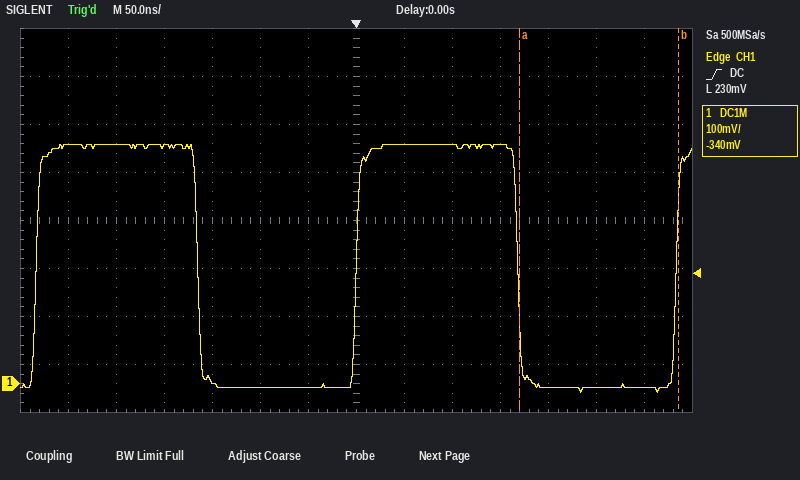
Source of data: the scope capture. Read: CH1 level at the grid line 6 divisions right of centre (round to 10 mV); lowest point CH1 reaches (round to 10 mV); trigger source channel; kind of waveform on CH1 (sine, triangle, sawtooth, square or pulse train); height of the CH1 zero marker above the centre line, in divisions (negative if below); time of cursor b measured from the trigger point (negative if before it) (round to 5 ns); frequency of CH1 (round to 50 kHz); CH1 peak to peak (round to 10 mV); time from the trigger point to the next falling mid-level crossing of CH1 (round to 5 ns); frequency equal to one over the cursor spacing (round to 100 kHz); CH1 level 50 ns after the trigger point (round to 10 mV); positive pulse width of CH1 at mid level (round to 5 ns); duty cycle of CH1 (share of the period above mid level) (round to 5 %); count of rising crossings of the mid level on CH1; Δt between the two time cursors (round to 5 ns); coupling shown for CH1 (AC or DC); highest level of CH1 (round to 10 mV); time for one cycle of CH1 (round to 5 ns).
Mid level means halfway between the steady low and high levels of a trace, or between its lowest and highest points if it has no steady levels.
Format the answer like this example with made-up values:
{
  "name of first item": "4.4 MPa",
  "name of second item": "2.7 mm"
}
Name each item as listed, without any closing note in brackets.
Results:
{
  "CH1 level at the grid line 6 divisions right of centre": "-10 mV",
  "lowest point CH1 reaches": "-20 mV",
  "trigger source channel": "CH1",
  "kind of waveform on CH1": "square",
  "height of the CH1 zero marker above the centre line, in divisions": "-3.4 div",
  "time of cursor b measured from the trigger point (negative if before it)": "+335 ns",
  "frequency of CH1": "3.00 MHz",
  "CH1 peak to peak": "520 mV",
  "time from the trigger point to the next falling mid-level crossing of CH1": "170 ns",
  "frequency equal to one over the cursor spacing": "6.1 MHz",
  "CH1 level 50 ns after the trigger point": "500 mV",
  "positive pulse width of CH1 at mid level": "170 ns",
  "duty cycle of CH1 (share of the period above mid level)": "50 %",
  "count of rising crossings of the mid level on CH1": "3",
  "Δt between the two time cursors": "165 ns",
  "coupling shown for CH1": "DC",
  "highest level of CH1": "500 mV",
  "time for one cycle of CH1": "335 ns"
}
